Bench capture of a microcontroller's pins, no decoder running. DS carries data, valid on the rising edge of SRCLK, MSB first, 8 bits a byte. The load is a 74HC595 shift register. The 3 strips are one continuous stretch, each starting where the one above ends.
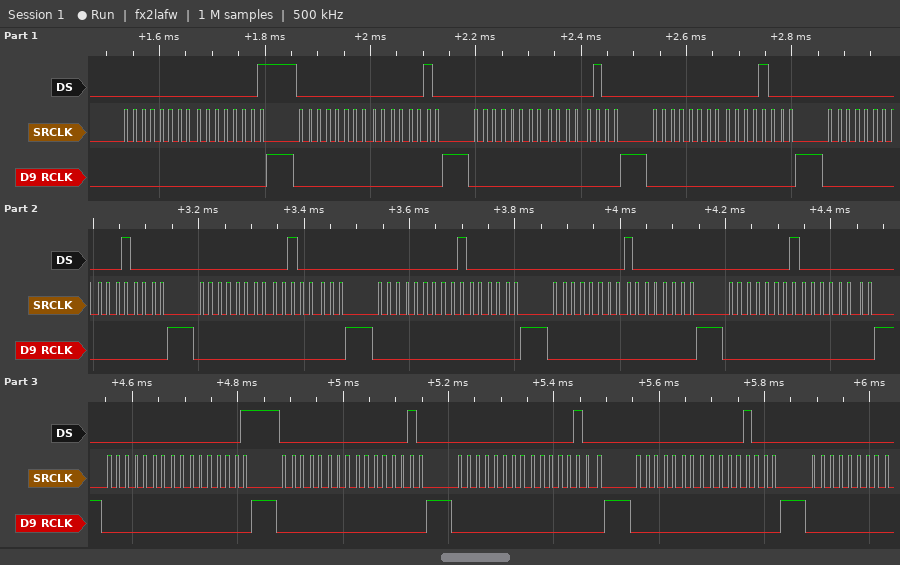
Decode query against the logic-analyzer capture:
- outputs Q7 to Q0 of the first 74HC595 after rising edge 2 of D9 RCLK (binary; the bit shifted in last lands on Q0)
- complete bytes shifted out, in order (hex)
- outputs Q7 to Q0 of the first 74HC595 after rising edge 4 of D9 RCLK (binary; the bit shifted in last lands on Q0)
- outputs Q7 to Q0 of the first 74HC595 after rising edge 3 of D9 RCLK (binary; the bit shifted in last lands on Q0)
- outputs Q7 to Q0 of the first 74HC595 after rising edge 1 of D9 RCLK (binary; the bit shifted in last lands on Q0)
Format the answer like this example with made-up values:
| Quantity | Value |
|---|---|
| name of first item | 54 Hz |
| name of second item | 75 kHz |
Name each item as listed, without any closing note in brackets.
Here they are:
| Quantity | Value |
|---|---|
| outputs Q7 to Q0 of the first 74HC595 after rising edge 2 of D9 RCLK | 00000010 |
| complete bytes shifted out, in order | 00 01 00 02 00 04 00 08 00 10 00 20 00 40 00 80 01 00 00 01 00 02 00 04 00 08 00 |
| outputs Q7 to Q0 of the first 74HC595 after rising edge 4 of D9 RCLK | 00001000 |
| outputs Q7 to Q0 of the first 74HC595 after rising edge 3 of D9 RCLK | 00000100 |
| outputs Q7 to Q0 of the first 74HC595 after rising edge 1 of D9 RCLK | 00000001 |
